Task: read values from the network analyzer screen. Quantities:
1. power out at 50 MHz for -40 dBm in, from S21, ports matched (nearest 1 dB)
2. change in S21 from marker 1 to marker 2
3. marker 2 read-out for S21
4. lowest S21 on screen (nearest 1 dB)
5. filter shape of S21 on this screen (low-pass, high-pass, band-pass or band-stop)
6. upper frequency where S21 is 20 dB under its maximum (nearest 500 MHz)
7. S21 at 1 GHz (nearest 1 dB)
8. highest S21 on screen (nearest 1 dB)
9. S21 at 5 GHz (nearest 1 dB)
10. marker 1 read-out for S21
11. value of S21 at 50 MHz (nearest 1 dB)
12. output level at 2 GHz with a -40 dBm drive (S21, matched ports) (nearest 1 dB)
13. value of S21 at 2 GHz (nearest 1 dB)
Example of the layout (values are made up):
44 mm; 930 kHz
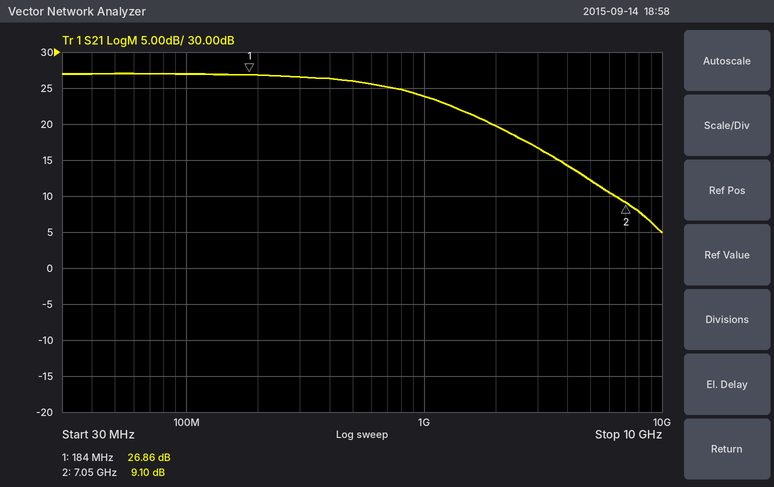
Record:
-13 dBm; -17.76 dB; 9.10 dB; 5 dB; low-pass; 8.5 GHz; 24 dB; 27 dB; 12 dB; 26.86 dB; 27 dB; -20 dBm; 20 dB
